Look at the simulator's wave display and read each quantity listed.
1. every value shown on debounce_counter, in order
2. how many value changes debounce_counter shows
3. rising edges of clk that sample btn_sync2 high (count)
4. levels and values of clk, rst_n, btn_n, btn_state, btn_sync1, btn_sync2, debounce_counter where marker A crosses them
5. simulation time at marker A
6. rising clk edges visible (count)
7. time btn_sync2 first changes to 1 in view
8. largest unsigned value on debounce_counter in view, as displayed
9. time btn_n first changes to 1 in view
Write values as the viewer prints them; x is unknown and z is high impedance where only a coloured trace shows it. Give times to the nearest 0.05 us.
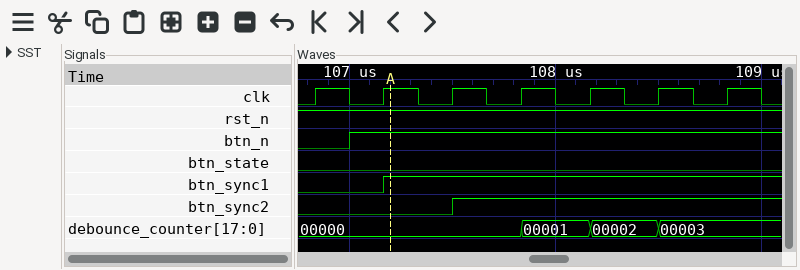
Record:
00000, 00001, 00002, 00003
3
4
clk=1, rst_n=1, btn_n=1, btn_state=0, btn_sync1=1, btn_sync2=0, debounce_counter=00000
107.2 us
7
107.5 us
00003
107 us
